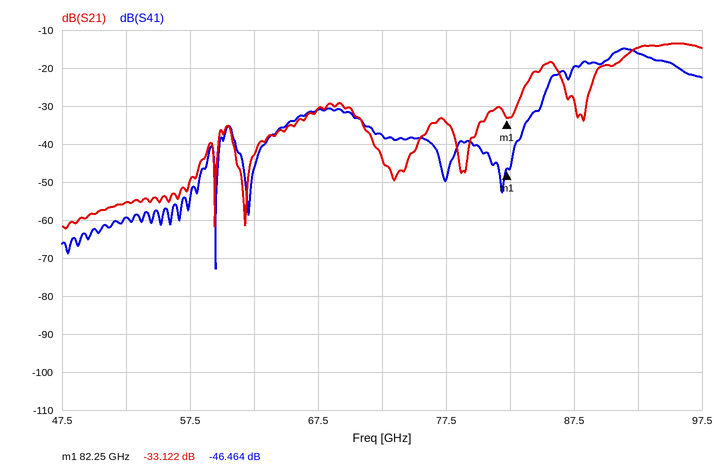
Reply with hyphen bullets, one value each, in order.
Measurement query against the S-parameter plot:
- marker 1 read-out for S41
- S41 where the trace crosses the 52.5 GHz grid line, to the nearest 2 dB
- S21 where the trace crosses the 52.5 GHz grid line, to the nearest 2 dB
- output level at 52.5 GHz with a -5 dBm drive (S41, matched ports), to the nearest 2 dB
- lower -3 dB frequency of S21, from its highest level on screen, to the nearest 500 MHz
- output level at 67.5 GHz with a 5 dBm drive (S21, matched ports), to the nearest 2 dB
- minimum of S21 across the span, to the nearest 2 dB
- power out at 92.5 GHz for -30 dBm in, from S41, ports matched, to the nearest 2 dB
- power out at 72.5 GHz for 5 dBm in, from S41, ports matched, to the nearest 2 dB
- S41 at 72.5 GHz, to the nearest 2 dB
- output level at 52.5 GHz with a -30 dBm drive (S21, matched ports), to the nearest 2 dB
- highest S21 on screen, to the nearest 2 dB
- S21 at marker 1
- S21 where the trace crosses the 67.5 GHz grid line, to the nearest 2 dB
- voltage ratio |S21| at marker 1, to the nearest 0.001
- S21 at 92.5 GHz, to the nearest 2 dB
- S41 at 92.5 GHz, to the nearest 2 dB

- -46.464 dB
- -60 dB
- -56 dB
- -64 dBm
- 91.5 GHz
- -26 dBm
- -62 dB
- -46 dBm
- -32 dBm
- -38 dB
- -86 dBm
- -14 dB
- -33.122 dB
- -30 dB
- 0.022
- -14 dB
- -16 dB
